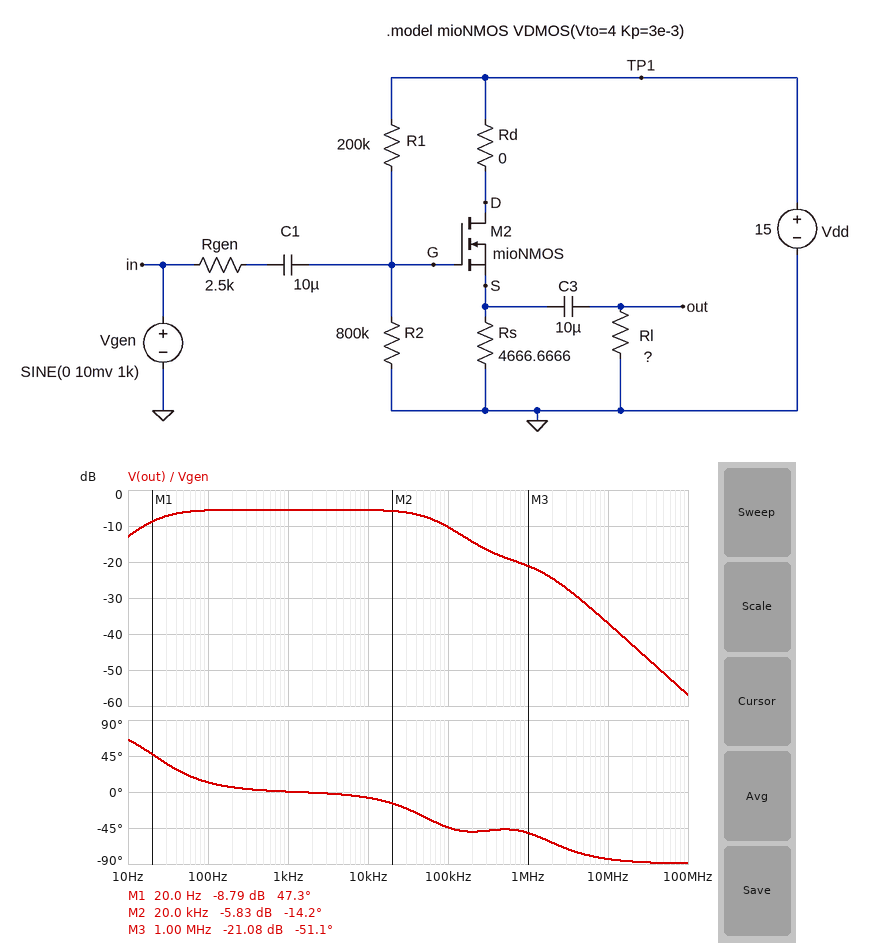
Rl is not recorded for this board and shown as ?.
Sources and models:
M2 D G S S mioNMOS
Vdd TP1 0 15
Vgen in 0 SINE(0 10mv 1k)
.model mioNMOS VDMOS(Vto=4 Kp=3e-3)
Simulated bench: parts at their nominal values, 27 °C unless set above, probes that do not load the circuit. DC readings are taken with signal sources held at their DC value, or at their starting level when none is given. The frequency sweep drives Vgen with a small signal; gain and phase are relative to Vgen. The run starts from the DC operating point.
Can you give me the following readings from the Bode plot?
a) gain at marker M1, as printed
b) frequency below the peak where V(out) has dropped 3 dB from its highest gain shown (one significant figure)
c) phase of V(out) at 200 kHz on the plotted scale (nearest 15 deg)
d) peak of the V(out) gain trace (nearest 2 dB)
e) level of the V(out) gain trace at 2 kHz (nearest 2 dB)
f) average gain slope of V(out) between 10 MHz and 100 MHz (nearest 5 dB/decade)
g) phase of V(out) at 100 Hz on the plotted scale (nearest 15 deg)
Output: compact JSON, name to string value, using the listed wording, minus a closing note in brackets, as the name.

{"gain at marker M1, as printed": "-8.79 dB", "frequency below the peak where V(out) has dropped 3 dB from its highest gain shown": "20 Hz", "phase of V(out) at 200 kHz on the plotted scale": "-45 deg", "peak of the V(out) gain trace": "-6 dB", "level of the V(out) gain trace at 2 kHz": "-6 dB", "average gain slope of V(out) between 10 MHz and 100 MHz": "-20 dB/decade", "phase of V(out) at 100 Hz on the plotted scale": "15 deg"}
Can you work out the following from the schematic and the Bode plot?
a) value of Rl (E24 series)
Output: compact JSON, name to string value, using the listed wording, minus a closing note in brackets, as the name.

{"value of Rl": "430 Ω"}
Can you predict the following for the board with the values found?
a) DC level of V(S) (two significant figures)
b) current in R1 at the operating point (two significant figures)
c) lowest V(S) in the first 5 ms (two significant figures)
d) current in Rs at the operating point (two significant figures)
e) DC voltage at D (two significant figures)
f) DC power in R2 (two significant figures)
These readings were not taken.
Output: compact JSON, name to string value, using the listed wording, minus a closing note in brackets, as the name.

{"DC level of V(S)": "7.0 V", "current in R1 at the operating point": "15 µA", "lowest V(S) in the first 5 ms": "7.0 V", "current in Rs at the operating point": "1.5 mA", "DC voltage at D": "15 V", "DC power in R2": "180 µW"}
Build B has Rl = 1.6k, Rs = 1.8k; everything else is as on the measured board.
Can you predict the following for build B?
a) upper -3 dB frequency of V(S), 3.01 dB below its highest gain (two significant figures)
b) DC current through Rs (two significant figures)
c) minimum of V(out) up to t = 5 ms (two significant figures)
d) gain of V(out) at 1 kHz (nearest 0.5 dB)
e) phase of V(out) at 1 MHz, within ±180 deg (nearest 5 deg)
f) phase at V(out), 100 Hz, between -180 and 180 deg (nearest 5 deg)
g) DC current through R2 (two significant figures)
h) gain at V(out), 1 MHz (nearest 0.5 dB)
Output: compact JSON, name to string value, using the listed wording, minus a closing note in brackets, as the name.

{"upper -3 dB frequency of V(S), 3.01 dB below its highest gain": "88 kHz", "DC current through Rs": "3.6 mA", "minimum of V(out) up to t = 5 ms": "-7.9 mV", "gain of V(out) at 1 kHz": "-2.0 dB", "phase of V(out) at 1 MHz, within ±180 deg": "-70 deg", "phase at V(out), 100 Hz, between -180 and 180 deg": "5 deg", "DC current through R2": "15 µA", "gain at V(out), 1 MHz": "-18.5 dB"}
